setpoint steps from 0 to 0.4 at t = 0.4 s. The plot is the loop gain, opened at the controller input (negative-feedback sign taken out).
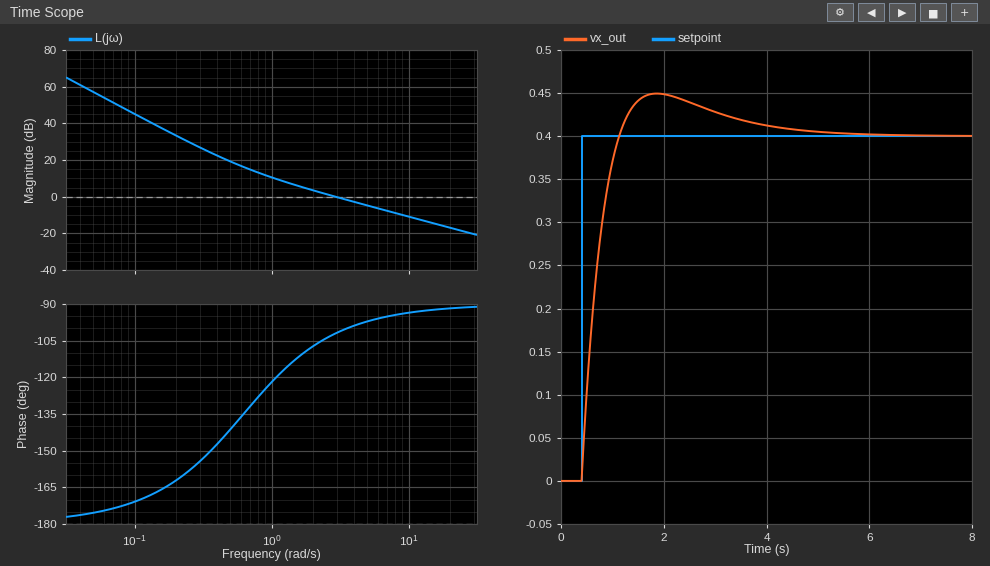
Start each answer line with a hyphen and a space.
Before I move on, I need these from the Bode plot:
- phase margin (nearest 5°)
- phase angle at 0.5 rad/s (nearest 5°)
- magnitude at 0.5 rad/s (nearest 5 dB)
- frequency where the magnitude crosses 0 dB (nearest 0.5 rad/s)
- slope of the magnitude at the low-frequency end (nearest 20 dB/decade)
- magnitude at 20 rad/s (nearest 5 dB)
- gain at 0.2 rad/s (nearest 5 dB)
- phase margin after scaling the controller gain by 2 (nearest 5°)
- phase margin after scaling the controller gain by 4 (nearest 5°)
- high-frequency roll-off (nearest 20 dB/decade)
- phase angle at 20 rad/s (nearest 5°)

- 80°
- -140°
- 20 dB
- 3.0 rad/s
- -40 dB/decade
- -15 dB
- 35 dB
- 85°
- 85°
- -20 dB/decade
- -90°
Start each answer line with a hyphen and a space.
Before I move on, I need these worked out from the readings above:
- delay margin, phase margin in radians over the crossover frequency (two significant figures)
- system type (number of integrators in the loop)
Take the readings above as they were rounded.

- 0.47 s
- 2
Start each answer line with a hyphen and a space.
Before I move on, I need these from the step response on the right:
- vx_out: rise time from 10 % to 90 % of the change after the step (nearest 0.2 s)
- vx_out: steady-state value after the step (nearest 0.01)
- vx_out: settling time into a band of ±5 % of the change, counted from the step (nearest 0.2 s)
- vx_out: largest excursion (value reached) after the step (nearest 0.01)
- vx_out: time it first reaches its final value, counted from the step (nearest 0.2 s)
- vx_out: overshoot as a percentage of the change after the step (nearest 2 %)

- 0.6 s
- 0.40
- 3.0 s
- 0.45
- 0.8 s
- 12 %
